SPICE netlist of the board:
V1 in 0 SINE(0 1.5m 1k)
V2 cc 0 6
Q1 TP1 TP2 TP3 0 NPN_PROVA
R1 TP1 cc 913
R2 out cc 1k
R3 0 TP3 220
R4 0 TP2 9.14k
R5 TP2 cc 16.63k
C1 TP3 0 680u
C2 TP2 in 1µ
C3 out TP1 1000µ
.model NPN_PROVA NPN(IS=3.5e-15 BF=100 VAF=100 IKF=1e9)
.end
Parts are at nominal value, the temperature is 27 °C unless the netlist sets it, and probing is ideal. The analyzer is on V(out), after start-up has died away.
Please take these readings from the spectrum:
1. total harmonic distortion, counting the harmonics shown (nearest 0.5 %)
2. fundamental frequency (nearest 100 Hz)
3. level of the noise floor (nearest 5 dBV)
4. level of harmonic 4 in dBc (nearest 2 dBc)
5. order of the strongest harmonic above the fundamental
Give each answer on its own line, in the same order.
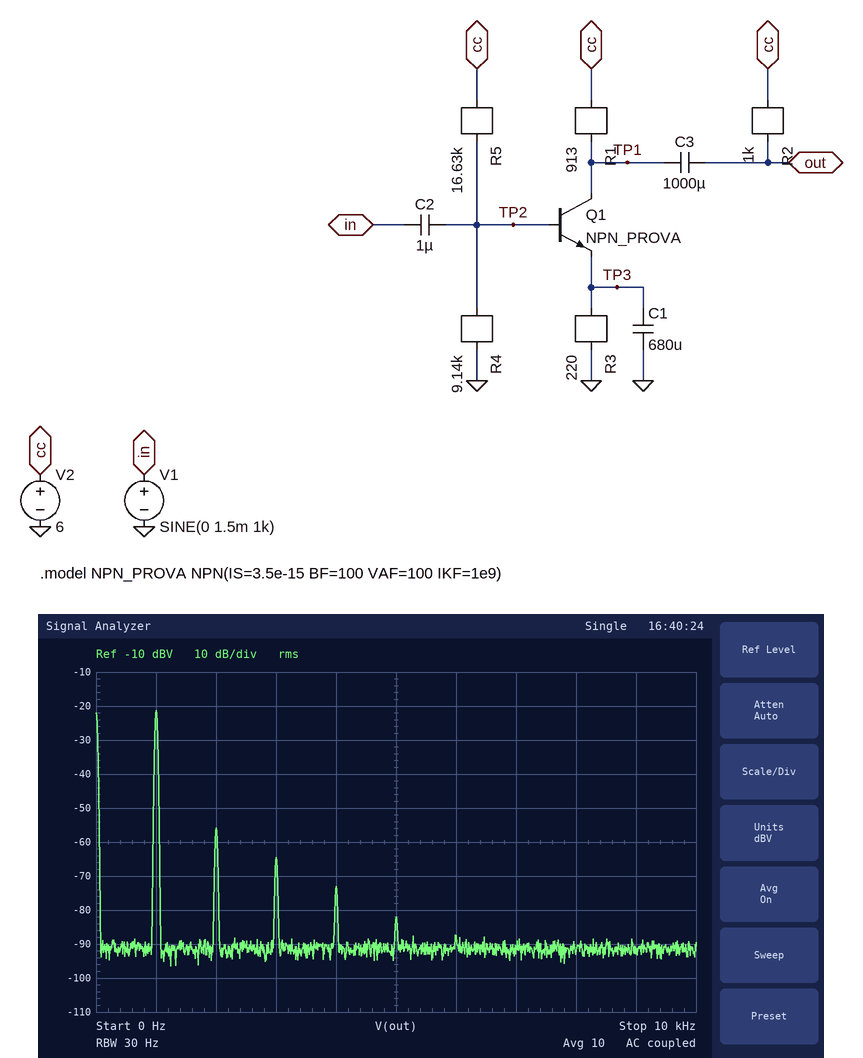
2.0 %
1.0 kHz
-90 dBV
-52 dBc
2
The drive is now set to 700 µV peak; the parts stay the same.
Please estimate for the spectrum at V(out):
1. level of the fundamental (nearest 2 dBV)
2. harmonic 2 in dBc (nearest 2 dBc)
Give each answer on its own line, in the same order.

-28 dBV
-44 dBc
